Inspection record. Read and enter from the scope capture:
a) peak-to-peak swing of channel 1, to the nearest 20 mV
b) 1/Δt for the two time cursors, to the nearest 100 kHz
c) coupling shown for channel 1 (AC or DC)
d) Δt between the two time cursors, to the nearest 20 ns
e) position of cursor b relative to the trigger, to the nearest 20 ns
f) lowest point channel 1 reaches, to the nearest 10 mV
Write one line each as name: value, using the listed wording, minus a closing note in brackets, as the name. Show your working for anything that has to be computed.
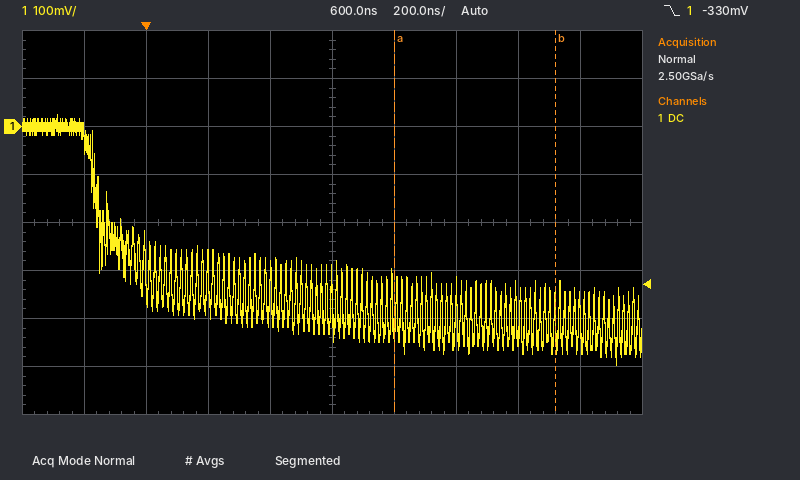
peak-to-peak swing of channel 1, to the nearest 20 mV: 520 mV
1/Δt for the two time cursors, to the nearest 100 kHz: 1 / 520 ns ≈ 1.9 MHz
coupling shown for channel 1: DC
Δt between the two time cursors, to the nearest 20 ns: 520 ns
position of cursor b relative to the trigger, to the nearest 20 ns: +1.32 µs
lowest point channel 1 reaches, to the nearest 10 mV: -500 mV
